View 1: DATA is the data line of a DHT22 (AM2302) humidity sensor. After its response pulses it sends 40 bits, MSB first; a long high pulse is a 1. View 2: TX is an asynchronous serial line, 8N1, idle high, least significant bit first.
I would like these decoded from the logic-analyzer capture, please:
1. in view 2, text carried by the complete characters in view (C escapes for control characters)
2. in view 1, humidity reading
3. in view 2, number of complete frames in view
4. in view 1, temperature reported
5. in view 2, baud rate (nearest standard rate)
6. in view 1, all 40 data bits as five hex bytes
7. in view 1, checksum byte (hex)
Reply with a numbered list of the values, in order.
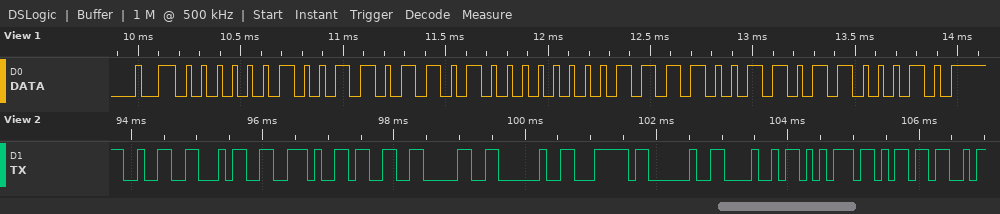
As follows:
1. "24.30 | Hum"
2. 62.1 %
3. 11
4. 24.3 °C
5. 9600 baud
6. 02 6D 00 F3 62
7. 0x62
